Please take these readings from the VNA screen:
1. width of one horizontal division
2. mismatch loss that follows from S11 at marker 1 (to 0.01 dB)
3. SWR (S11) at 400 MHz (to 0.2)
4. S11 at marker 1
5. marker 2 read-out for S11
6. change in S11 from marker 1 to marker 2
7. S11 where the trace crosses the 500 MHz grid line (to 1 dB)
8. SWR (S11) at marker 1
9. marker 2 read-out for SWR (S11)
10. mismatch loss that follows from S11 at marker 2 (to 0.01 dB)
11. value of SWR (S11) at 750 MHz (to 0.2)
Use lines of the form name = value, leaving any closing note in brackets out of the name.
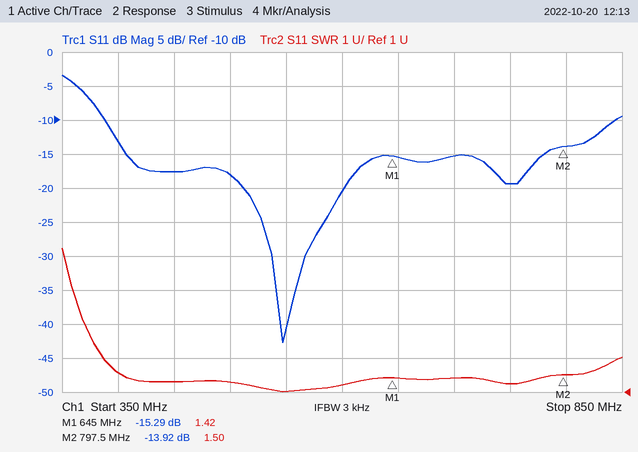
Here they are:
width of one horizontal division = 50 MHz
mismatch loss that follows from S11 at marker 1 = 0.13 dB
SWR (S11) at 400 MHz = 1.6
S11 at marker 1 = -15.29 dB
marker 2 read-out for S11 = -13.92 dB
change in S11 from marker 1 to marker 2 = 1.37 dB
S11 where the trace crosses the 500 MHz grid line = -18 dB
SWR (S11) at marker 1 = 1.42
marker 2 read-out for SWR = 1.50
mismatch loss that follows from S11 at marker 2 = 0.18 dB
value of SWR (S11) at 750 MHz = 1.2
